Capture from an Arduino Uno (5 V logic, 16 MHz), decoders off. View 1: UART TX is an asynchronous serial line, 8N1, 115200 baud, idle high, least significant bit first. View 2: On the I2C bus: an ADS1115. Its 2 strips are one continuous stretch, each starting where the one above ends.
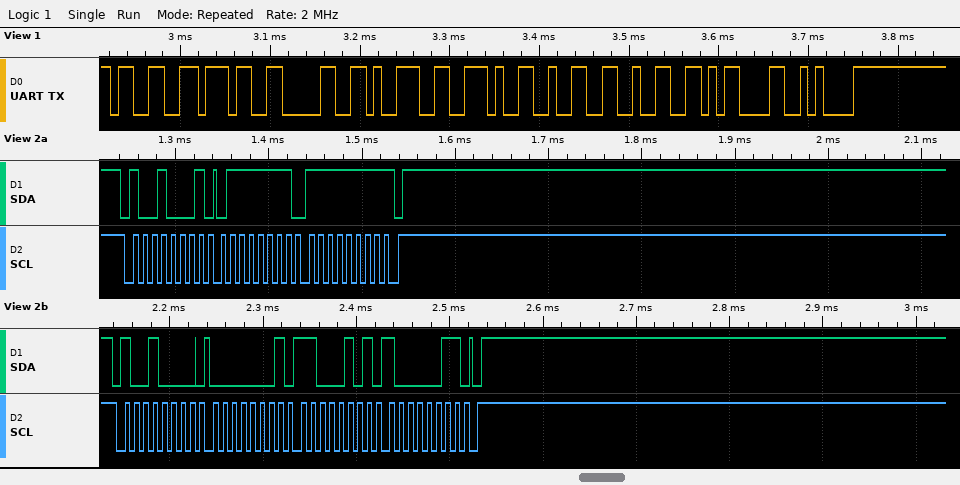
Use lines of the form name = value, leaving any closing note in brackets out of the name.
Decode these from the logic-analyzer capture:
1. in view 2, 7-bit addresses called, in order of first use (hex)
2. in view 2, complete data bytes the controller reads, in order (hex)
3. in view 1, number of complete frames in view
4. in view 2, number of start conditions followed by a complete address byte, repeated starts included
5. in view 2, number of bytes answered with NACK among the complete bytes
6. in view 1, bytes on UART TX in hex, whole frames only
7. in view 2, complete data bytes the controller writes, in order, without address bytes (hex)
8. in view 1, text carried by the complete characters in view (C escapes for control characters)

in view 2, 7-bit addresses called, in order of first use = 0x48
in view 2, complete data bytes the controller reads, in order = 7F FF
in view 1, number of complete frames in view = 9
in view 2, number of start conditions followed by a complete address byte, repeated starts included = 2
in view 2, number of bytes answered with NACK among the complete bytes = 1
in view 1, bytes on UART TX in hex, whole frames only = 33 37 30 39 2E 32 32 0D 0A
in view 2, complete data bytes the controller writes, in order, without address bytes = 01 C5 83
in view 1, text carried by the complete characters in view = "3709.22\r\n"
